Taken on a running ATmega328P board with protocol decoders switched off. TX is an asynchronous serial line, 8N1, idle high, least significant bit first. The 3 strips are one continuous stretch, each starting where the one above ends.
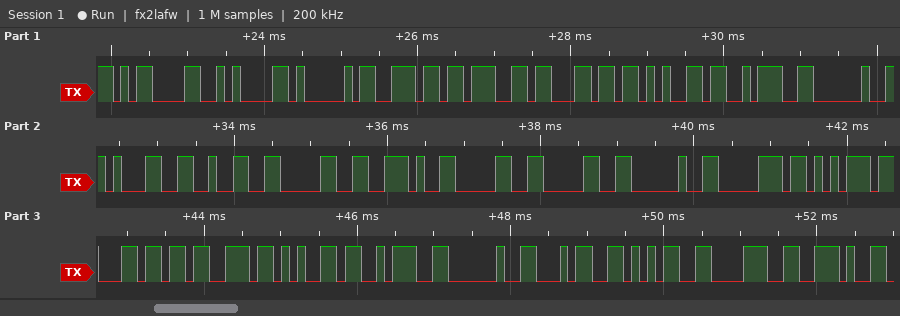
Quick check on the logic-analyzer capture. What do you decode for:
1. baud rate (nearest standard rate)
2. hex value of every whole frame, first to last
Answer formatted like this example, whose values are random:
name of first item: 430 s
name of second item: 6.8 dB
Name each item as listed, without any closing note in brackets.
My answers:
baud rate: 9600 baud
hex value of every whole frame, first to last: 0D 0A 41 6E 67 6C 65 3A 20 31 32 30 2E 30 30 20 70 75 6C 73 65 3A 20 34 35 38 2E
